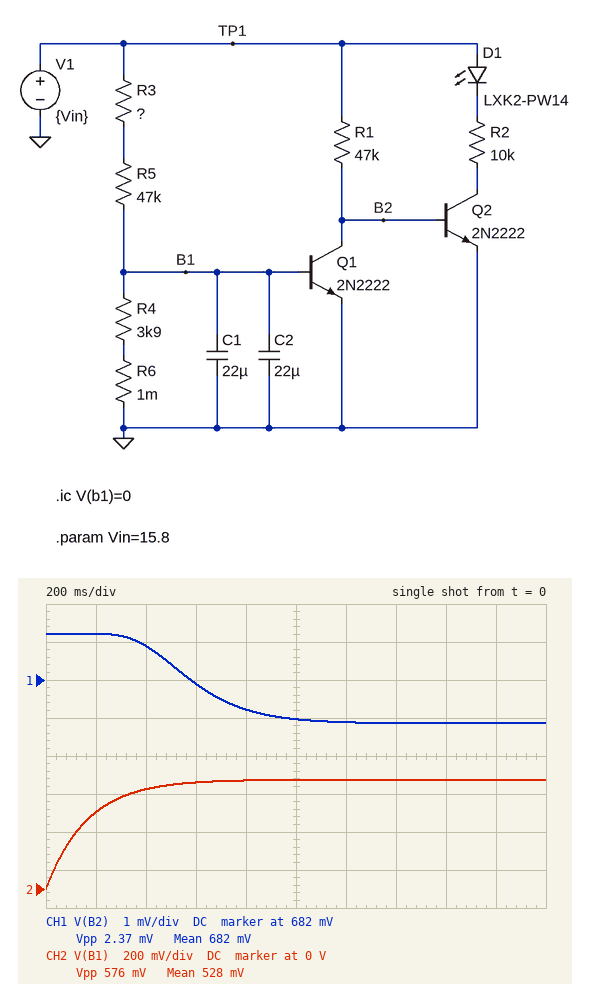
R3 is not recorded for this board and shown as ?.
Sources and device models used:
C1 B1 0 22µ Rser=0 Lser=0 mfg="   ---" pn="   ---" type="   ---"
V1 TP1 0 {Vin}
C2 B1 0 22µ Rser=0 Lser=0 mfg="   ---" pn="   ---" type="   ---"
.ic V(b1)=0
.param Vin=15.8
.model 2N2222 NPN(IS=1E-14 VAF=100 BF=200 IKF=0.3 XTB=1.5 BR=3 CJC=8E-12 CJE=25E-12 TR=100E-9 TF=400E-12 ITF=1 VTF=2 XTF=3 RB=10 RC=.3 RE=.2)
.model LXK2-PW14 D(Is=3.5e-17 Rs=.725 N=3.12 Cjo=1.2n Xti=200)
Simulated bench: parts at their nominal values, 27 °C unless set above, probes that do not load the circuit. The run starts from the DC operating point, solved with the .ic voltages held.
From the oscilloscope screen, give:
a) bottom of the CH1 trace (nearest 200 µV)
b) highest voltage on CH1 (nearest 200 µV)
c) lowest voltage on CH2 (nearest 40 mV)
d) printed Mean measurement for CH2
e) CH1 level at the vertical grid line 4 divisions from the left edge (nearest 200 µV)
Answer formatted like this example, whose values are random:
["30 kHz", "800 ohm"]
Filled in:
["680.8 mV", "683.2 mV", "0 V", "528 mV", "681.2 mV"]
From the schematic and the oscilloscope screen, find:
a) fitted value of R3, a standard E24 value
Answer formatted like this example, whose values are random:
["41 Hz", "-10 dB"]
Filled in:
["56 kΩ"]
